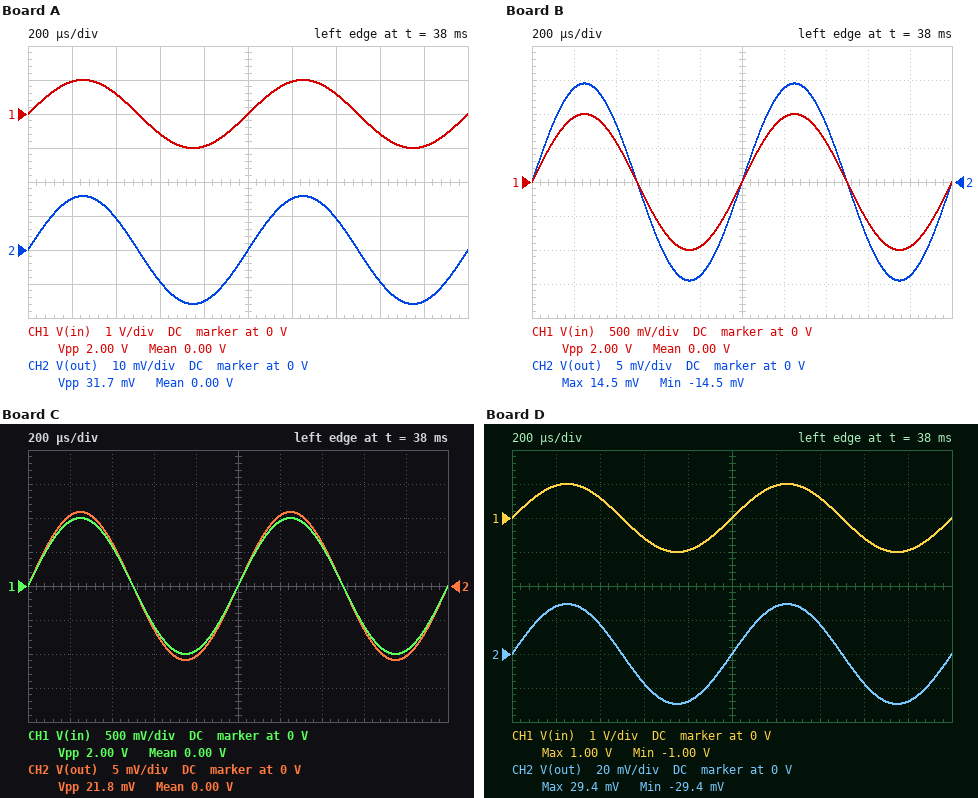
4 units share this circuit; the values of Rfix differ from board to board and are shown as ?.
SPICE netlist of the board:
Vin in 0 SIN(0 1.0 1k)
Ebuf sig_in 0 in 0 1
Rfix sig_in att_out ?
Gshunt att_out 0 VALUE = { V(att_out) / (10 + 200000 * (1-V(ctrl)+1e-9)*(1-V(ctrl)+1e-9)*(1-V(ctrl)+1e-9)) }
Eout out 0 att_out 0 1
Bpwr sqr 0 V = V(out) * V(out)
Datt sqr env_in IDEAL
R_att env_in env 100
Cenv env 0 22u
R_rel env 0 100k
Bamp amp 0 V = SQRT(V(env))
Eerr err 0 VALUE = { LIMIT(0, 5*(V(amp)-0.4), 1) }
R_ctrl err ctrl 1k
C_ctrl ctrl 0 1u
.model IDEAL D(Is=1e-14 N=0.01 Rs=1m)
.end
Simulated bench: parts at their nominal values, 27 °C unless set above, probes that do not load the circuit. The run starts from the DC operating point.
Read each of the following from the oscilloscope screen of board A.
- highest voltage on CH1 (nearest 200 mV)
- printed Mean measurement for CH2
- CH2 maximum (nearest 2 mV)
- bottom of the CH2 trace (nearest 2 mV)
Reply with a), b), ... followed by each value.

a) 1.0 V
b) 0.00 V
c) 16 mV
d) -16 mV
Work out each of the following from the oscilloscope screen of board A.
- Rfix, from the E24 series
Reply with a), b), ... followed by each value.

a) 620 Ω
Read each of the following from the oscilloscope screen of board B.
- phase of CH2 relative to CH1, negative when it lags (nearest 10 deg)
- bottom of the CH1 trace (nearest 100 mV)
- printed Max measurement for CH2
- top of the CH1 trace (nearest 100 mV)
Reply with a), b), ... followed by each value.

a) 0 deg
b) -1.0 V
c) 14.5 mV
d) 1.0 V
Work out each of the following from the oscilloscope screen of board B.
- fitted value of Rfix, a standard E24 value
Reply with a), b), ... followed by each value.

a) 680 Ω
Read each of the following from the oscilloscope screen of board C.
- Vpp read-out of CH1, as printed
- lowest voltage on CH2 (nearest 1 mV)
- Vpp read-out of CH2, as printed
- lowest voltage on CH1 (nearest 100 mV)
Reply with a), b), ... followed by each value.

a) 2.00 V
b) -11 mV
c) 21.8 mV
d) -1.0 V
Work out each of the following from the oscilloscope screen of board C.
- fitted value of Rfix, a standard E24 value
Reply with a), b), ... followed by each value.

a) 910 Ω
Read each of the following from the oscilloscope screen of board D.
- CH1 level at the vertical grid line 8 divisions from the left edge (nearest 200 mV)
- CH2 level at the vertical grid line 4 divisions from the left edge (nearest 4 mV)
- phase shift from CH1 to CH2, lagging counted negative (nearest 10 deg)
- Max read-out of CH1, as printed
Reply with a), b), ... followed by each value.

a) -600 mV
b) -28 mV
c) 0 deg
d) 1.00 V
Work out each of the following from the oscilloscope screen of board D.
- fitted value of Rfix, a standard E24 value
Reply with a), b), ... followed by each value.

a) 330 Ω
